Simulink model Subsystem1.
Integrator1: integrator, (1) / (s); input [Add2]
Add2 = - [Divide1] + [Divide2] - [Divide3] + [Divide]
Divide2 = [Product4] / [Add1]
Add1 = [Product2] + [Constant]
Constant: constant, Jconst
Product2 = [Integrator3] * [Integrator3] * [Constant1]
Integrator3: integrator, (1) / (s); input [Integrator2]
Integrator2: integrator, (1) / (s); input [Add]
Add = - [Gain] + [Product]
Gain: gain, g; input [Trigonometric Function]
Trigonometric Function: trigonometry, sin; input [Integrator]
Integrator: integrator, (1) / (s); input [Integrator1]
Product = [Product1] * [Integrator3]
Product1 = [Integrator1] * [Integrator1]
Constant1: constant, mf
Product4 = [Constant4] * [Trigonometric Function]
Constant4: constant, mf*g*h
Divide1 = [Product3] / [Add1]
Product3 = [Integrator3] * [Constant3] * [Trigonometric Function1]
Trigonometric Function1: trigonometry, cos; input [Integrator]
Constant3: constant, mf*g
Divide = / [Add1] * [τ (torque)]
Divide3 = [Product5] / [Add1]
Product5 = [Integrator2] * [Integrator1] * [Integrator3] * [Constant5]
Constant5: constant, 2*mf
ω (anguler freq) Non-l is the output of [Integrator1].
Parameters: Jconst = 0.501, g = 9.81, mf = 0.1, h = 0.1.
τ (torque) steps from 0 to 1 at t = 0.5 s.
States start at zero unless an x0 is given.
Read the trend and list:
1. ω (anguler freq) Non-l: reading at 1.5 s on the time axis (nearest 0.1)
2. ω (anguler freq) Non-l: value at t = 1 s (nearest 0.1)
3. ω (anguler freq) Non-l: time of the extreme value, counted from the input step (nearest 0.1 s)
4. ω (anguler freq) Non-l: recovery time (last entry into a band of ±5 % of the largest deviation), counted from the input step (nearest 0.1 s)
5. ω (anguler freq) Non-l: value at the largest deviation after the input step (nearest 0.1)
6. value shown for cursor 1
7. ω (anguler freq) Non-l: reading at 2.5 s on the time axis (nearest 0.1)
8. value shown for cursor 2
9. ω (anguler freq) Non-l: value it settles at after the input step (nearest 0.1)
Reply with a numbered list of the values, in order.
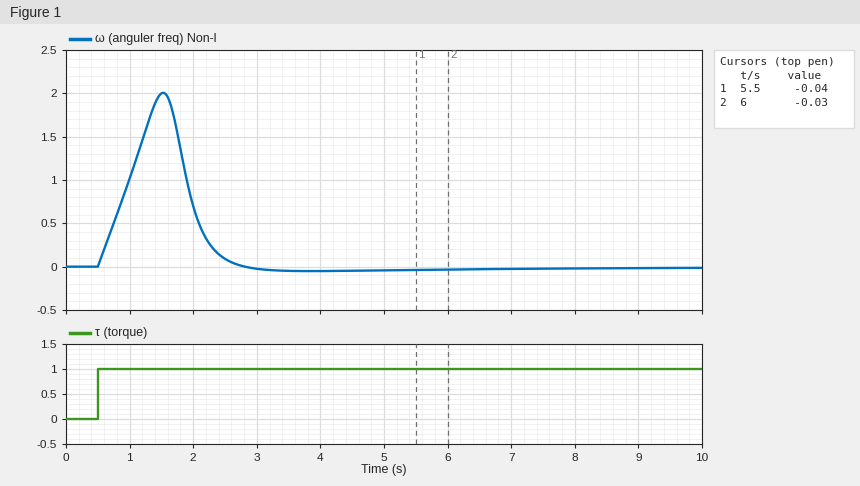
1. 2.0
2. 1.0
3. 1.0 s
4. 2.0 s
5. 2.0
6. -0.04
7. 0.1
8. -0.03
9. 0.0
